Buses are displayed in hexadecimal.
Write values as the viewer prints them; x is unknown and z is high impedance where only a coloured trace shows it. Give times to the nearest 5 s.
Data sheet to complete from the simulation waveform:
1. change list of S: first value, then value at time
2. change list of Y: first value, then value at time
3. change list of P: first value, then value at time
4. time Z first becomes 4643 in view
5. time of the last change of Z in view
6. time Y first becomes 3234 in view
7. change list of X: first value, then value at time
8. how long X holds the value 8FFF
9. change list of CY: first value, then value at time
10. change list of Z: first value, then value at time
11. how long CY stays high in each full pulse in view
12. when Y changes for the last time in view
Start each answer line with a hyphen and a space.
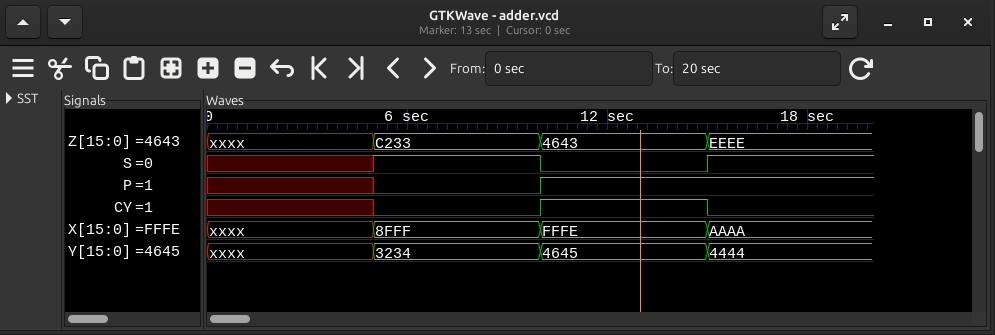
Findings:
- x, 1 at 5 s, 0 at 10 s, 1 at 15 s
- xxxx, 3234 at 5 s, 4645 at 10 s, 4444 at 15 s
- x, 0 at 5 s, 1 at 10 s
- 10 s
- 15 s
- 5 s
- xxxx, 8FFF at 5 s, FFFE at 10 s, AAAA at 15 s
- 5 s
- x, 0 at 5 s, 1 at 10 s, 0 at 15 s
- xxxx, C233 at 5 s, 4643 at 10 s, EEEE at 15 s
- 5 s
- 15 s
